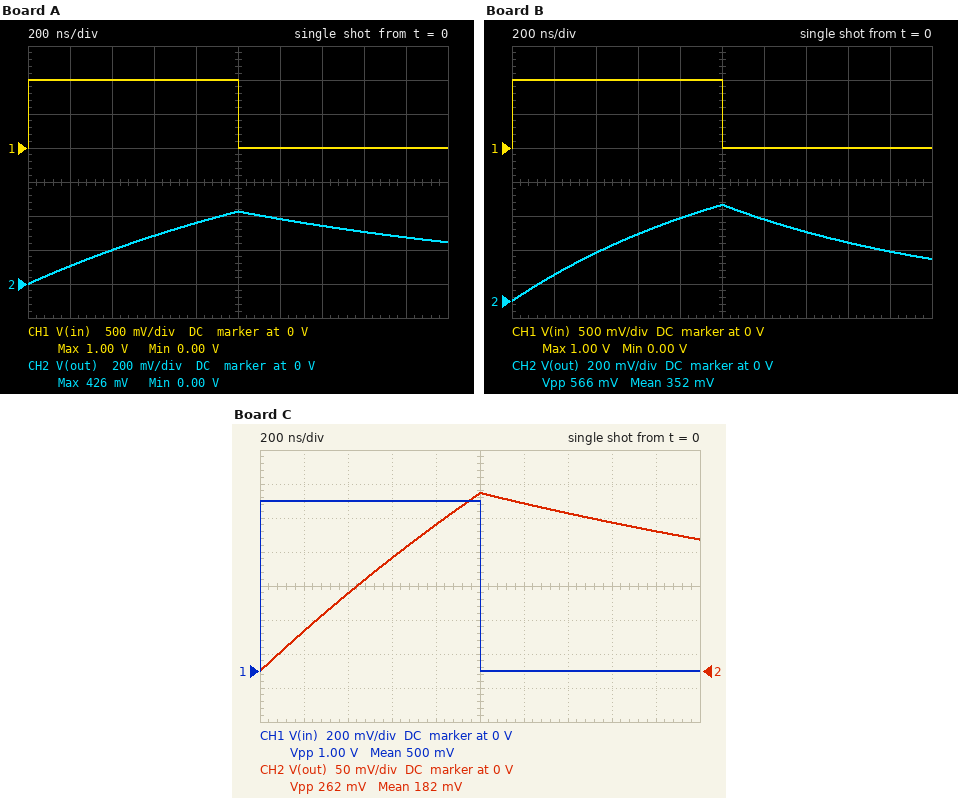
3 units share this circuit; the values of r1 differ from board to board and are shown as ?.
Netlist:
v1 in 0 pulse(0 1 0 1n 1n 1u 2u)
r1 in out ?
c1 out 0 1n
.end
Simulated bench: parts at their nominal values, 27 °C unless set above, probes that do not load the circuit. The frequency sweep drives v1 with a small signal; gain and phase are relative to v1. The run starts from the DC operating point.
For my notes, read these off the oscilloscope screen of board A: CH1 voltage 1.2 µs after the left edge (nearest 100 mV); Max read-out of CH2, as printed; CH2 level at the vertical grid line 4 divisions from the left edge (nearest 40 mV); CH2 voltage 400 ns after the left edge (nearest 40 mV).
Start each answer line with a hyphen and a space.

- 0 V
- 426 mV
- 360 mV
- 200 mV
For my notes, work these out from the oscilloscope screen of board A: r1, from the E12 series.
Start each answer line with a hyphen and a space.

- 1.8 kΩ
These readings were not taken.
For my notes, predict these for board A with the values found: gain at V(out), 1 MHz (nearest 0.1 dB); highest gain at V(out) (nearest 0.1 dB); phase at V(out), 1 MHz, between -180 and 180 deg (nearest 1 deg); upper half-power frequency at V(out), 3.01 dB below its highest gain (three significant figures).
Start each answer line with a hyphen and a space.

- -21.1 dB
- 0 dB
- -85 deg
- 88.4 kHz
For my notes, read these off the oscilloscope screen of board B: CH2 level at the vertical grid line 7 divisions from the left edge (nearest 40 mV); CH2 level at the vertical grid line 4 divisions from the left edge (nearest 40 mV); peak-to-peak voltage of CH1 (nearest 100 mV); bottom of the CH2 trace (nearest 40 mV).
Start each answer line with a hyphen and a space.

- 400 mV
- 480 mV
- 1.0 V
- 0 V
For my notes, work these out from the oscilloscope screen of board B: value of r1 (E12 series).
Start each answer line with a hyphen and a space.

- 1.2 kΩ
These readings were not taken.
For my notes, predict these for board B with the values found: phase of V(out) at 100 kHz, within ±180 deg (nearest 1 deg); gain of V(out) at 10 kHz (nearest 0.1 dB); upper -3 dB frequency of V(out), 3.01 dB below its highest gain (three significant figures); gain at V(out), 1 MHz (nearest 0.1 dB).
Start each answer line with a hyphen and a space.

- -37 deg
- 0 dB
- 133 kHz
- -17.6 dB
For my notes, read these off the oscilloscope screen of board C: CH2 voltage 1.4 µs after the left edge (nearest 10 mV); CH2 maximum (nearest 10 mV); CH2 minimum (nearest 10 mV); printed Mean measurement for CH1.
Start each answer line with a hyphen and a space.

- 230 mV
- 260 mV
- 0 V
- 500 mV
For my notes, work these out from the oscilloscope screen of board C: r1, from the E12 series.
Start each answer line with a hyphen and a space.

- 3.3 kΩ
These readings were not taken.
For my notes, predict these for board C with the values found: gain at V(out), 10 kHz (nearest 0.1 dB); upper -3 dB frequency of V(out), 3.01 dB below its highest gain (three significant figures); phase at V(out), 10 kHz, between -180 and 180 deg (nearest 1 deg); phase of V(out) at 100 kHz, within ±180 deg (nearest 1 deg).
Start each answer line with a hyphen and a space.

- -0.2 dB
- 48.2 kHz
- -12 deg
- -64 deg
